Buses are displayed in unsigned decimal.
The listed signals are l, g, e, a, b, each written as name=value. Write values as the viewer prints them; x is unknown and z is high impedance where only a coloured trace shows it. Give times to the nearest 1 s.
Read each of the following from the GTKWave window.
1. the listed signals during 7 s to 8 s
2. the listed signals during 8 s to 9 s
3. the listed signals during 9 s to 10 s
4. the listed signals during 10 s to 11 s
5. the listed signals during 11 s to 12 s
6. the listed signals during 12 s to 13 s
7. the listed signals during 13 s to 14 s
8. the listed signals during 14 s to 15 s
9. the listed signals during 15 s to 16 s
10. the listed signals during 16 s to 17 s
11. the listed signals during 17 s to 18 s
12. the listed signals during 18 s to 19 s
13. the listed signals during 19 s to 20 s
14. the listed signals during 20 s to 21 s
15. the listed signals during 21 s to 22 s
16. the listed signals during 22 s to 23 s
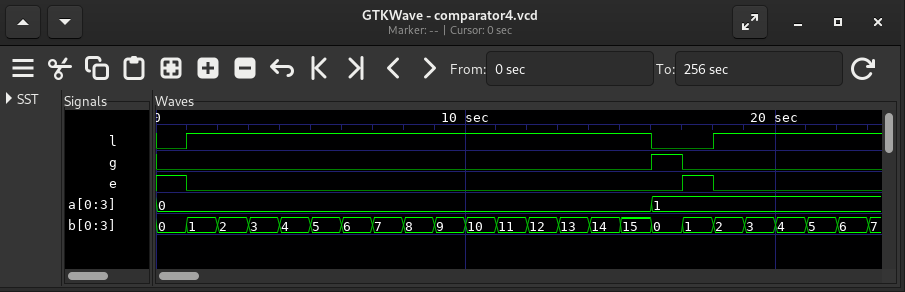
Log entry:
l=1, g=0, e=0, a=0, b=7
l=1, g=0, e=0, a=0, b=8
l=1, g=0, e=0, a=0, b=9
l=1, g=0, e=0, a=0, b=10
l=1, g=0, e=0, a=0, b=11
l=1, g=0, e=0, a=0, b=12
l=1, g=0, e=0, a=0, b=13
l=1, g=0, e=0, a=0, b=14
l=1, g=0, e=0, a=0, b=15
l=0, g=1, e=0, a=1, b=0
l=0, g=0, e=1, a=1, b=1
l=1, g=0, e=0, a=1, b=2
l=1, g=0, e=0, a=1, b=3
l=1, g=0, e=0, a=1, b=4
l=1, g=0, e=0, a=1, b=5
l=1, g=0, e=0, a=1, b=6
